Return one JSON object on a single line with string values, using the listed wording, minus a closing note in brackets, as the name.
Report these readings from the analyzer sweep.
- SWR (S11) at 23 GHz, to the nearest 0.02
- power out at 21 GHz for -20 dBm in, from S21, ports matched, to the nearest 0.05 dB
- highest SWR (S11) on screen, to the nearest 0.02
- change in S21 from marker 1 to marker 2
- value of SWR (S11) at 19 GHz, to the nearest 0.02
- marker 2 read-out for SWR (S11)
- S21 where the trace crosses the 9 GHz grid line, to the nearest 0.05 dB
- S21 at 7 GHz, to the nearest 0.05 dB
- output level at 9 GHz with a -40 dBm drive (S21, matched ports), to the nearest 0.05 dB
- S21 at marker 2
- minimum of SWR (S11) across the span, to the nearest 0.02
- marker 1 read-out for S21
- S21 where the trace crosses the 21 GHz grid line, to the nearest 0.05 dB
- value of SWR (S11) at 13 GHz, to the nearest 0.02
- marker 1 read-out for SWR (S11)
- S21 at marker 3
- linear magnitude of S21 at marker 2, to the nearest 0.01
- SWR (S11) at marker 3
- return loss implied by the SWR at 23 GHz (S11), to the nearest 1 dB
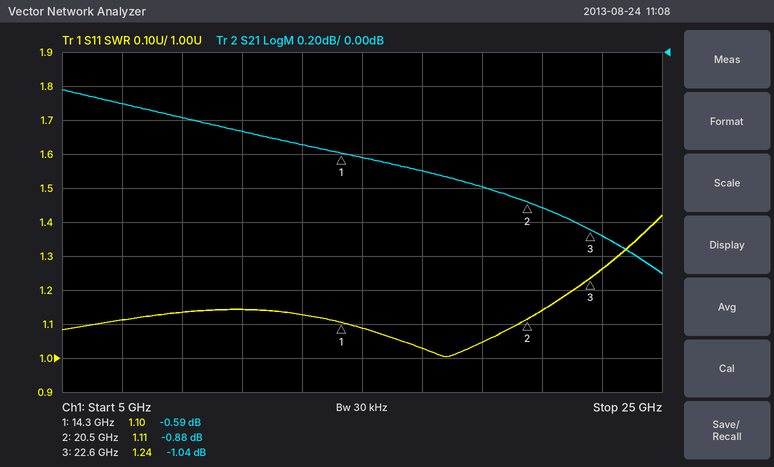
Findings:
{"SWR (S11) at 23 GHz, to the nearest 0.02": "1.26", "power out at 21 GHz for -20 dBm in, from S21, ports matched, to the nearest 0.05 dB": "-20.90 dBm", "highest SWR (S11) on screen, to the nearest 0.02": "1.42", "change in S21 from marker 1 to marker 2": "-0.29 dB", "value of SWR (S11) at 19 GHz, to the nearest 0.02": "1.04", "marker 2 read-out for SWR": "1.11", "S21 where the trace crosses the 9 GHz grid line, to the nearest 0.05 dB": "-0.40 dB", "S21 at 7 GHz, to the nearest 0.05 dB": "-0.30 dB", "output level at 9 GHz with a -40 dBm drive (S21, matched ports), to the nearest 0.05 dB": "-40.40 dBm", "S21 at marker 2": "-0.88 dB", "minimum of SWR (S11) across the span, to the nearest 0.02": "1.00", "marker 1 read-out for S21": "-0.59 dB", "S21 where the trace crosses the 21 GHz grid line, to the nearest 0.05 dB": "-0.90 dB", "value of SWR (S11) at 13 GHz, to the nearest 0.02": "1.12", "marker 1 read-out for SWR": "1.10", "S21 at marker 3": "-1.04 dB", "linear magnitude of S21 at marker 2, to the nearest 0.01": "0.90", "SWR (S11) at marker 3": "1.24", "return loss implied by the SWR at 23 GHz (S11), to the nearest 1 dB": "19 dB"}
